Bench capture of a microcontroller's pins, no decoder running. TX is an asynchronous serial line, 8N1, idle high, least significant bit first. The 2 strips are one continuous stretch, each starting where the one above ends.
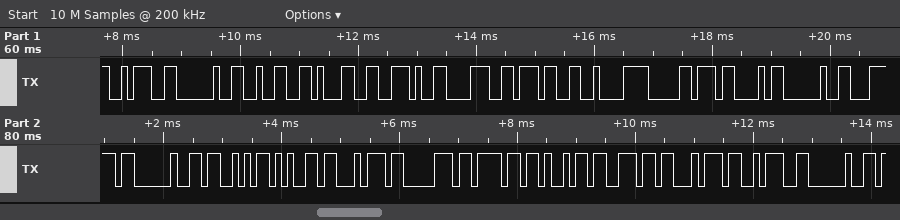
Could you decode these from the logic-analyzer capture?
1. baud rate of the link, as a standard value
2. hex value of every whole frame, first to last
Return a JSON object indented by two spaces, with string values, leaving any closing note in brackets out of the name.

{
  "baud rate of the link, as a standard value": "9600 baud",
  "hex value of every whole frame, first to last": "3A 20 32 31 2E 38 37 C2 B0 43 20 7C 20 53 65 74 70 6F 69 6E 74 3A 20"
}
